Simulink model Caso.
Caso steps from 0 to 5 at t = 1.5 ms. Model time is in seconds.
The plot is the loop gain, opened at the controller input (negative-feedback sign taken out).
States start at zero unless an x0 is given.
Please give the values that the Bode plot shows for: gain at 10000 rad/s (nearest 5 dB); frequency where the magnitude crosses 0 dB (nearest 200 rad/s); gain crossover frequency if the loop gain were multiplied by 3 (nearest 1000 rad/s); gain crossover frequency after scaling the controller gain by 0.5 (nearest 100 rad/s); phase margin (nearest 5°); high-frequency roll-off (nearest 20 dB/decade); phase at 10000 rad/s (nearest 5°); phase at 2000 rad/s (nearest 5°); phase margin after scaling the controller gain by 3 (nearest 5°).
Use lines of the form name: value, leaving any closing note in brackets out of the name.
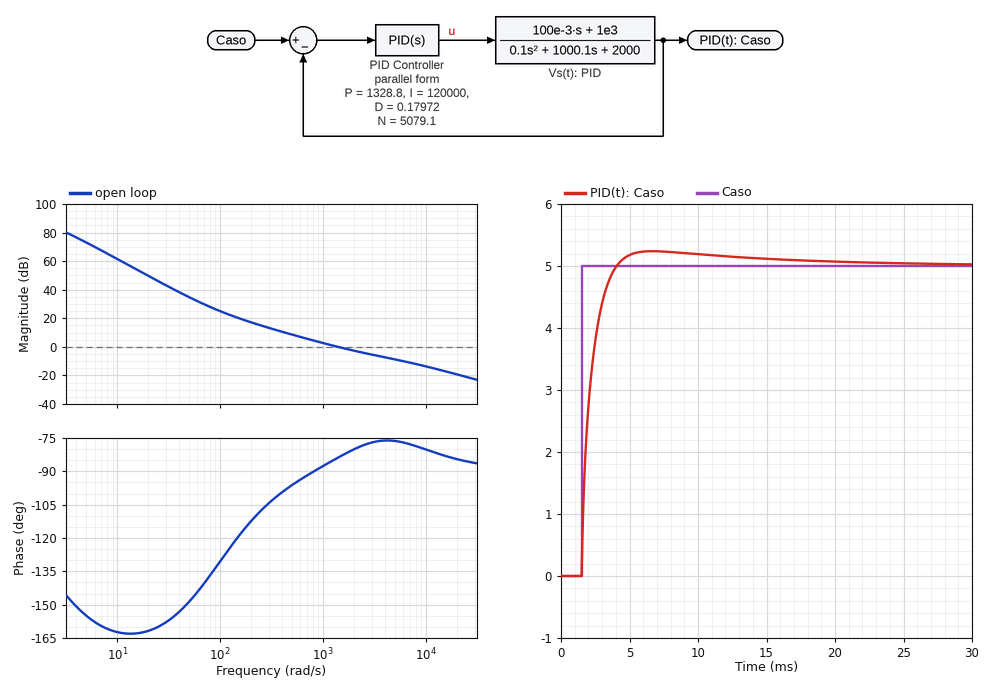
gain at 10000 rad/s: -15 dB
frequency where the magnitude crosses 0 dB: 1400 rad/s
gain crossover frequency if the loop gain were multiplied by 3: 6000 rad/s
gain crossover frequency after scaling the controller gain by 0.5: 700 rad/s
phase margin: 95°
high-frequency roll-off: -20 dB/decade
phase at 10000 rad/s: -80°
phase at 2000 rad/s: -80°
phase margin after scaling the controller gain by 3: 105°
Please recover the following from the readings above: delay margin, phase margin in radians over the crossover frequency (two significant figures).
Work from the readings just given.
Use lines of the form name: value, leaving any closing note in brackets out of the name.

delay margin, phase margin in radians over the crossover frequency: 0.0012 s
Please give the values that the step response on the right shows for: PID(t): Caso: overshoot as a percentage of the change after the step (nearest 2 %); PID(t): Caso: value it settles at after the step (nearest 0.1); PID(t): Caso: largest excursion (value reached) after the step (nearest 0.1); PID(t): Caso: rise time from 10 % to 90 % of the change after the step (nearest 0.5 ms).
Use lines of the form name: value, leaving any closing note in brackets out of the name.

PID(t): Caso: overshoot as a percentage of the change after the step: 4 %
PID(t): Caso: value it settles at after the step: 5.0
PID(t): Caso: largest excursion (value reached) after the step: 5.2
PID(t): Caso: rise time from 10 % to 90 % of the change after the step: 1.5 ms
